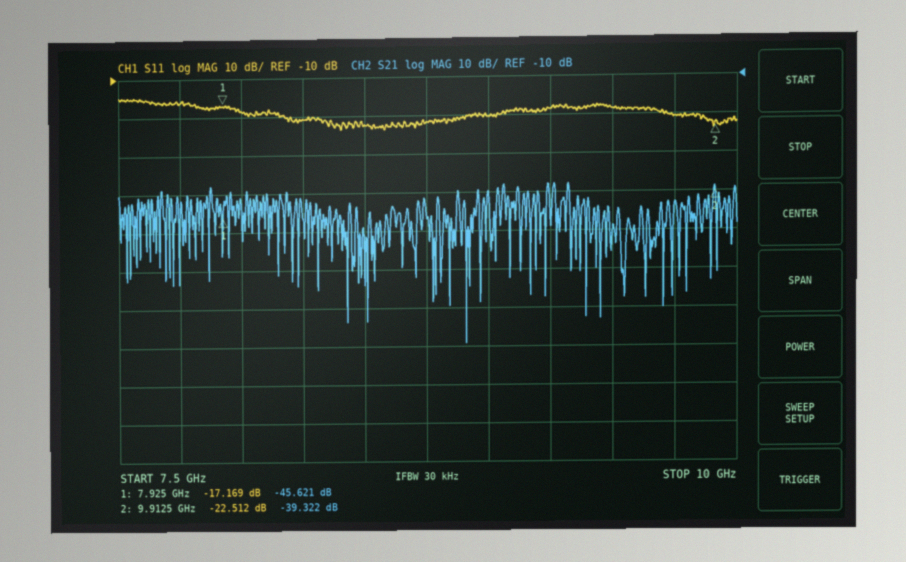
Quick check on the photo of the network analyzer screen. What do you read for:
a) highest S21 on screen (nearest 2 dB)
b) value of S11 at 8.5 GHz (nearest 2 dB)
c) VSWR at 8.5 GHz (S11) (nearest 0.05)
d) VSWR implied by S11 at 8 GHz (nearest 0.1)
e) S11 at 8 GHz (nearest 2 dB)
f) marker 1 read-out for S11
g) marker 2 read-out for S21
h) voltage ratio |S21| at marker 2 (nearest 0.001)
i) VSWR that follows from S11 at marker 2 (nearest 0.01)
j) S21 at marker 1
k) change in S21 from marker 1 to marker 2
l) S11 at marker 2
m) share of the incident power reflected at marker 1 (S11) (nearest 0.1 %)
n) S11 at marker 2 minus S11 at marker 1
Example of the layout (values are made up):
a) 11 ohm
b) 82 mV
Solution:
a) -38 dB
b) -22 dB
c) 1.15
d) 1.3
e) -18 dB
f) -17.169 dB
g) -39.322 dB
h) 0.011
i) 1.16
j) -45.621 dB
k) 6.299 dB
l) -22.512 dB
m) 1.9 %
n) -5.343 dB
